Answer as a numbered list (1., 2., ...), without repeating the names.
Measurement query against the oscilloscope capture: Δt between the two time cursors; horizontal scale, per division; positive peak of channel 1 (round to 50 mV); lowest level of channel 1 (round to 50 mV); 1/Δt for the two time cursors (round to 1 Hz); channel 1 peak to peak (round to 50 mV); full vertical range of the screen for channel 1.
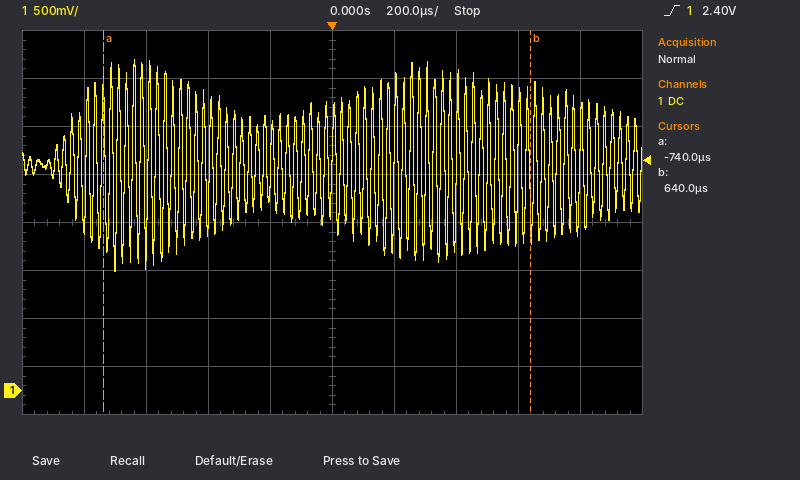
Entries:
1. 1.38 ms
2. 200 µs
3. 3.45 V
4. 1.25 V
5. 725 Hz
6. 2.20 V
7. 4 V
